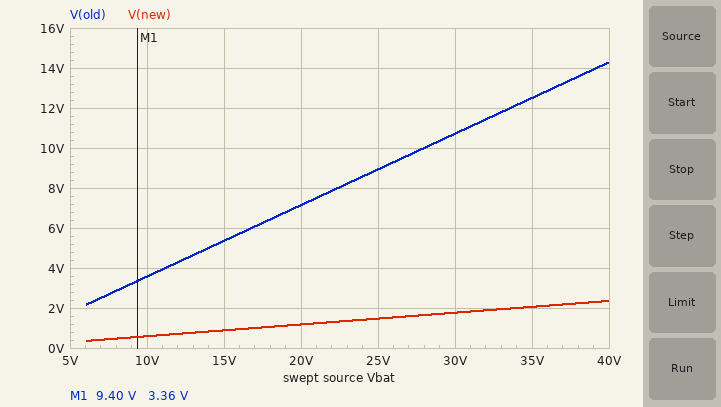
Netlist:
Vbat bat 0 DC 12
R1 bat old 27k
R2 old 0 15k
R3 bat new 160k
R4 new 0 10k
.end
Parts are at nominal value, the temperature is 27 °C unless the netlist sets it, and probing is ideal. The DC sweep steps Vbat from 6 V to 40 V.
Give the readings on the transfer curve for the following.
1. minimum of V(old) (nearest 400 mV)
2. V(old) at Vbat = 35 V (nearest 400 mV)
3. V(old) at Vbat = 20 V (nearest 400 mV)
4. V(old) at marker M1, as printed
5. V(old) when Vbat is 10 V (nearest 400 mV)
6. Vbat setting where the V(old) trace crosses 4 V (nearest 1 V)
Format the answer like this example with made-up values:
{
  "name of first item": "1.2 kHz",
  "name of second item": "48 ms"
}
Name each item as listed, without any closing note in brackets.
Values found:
{
  "minimum of V(old)": "2.0 V",
  "V(old) at Vbat = 35 V": "12.4 V",
  "V(old) at Vbat = 20 V": "7.2 V",
  "V(old) at marker M1, as printed": "3.36 V",
  "V(old) when Vbat is 10 V": "3.6 V",
  "Vbat setting where the V(old) trace crosses 4 V": "11 V"
}
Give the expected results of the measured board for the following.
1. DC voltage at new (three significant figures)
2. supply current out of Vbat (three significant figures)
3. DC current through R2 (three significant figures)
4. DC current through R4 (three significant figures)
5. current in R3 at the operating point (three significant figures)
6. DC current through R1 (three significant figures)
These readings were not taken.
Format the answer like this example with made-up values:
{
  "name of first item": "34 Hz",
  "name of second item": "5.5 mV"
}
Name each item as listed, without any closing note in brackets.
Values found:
{
  "DC voltage at new": "706 mV",
  "supply current out of Vbat": "356 µA",
  "DC current through R2": "286 µA",
  "DC current through R4": "70.6 µA",
  "current in R3 at the operating point": "70.6 µA",
  "DC current through R1": "286 µA"
}
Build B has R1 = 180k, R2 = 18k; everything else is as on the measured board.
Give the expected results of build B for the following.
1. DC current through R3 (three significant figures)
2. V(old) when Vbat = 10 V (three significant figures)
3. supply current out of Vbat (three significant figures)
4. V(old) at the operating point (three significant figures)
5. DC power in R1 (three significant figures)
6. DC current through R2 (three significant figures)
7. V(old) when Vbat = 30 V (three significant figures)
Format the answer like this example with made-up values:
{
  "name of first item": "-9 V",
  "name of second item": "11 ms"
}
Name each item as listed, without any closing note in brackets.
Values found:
{
  "DC current through R3": "70.6 µA",
  "V(old) when Vbat = 10 V": "909 mV",
  "supply current out of Vbat": "131 µA",
  "V(old) at the operating point": "1.09 V",
  "DC power in R1": "661 µW",
  "DC current through R2": "60.6 µA",
  "V(old) when Vbat = 30 V": "2.73 V"
}
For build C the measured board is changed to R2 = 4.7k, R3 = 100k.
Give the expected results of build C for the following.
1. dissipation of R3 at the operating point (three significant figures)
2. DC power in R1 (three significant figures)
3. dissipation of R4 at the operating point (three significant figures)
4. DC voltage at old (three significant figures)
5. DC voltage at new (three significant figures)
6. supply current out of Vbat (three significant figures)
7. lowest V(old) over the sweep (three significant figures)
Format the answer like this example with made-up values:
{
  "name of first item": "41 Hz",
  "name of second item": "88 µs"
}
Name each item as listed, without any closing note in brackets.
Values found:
{
  "dissipation of R3 at the operating point": "1.19 mW",
  "DC power in R1": "3.87 mW",
  "dissipation of R4 at the operating point": "119 µW",
  "DC voltage at old": "1.78 V",
  "DC voltage at new": "1.09 V",
  "supply current out of Vbat": "488 µA",
  "lowest V(old) over the sweep": "890 mV"
}
